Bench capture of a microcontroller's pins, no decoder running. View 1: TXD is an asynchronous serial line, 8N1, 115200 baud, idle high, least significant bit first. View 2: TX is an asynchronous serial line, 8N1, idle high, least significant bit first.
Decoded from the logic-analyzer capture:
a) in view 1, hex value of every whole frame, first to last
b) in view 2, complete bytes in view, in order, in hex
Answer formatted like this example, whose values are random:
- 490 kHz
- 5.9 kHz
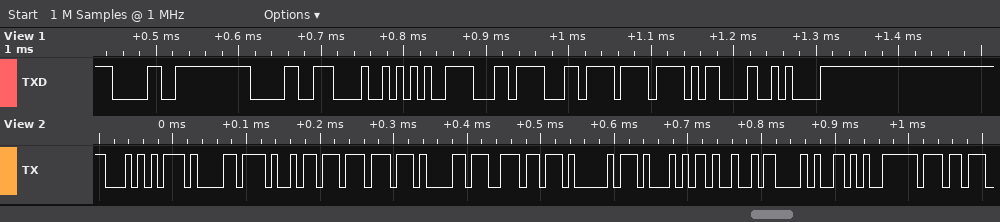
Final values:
- 0x30 0x30 0x48 0xE5 0xEC 0xEC 0xEF 0x0D 0x0A
- 54 61 69 77 61 6E 41 51 49 28 E5 B7
